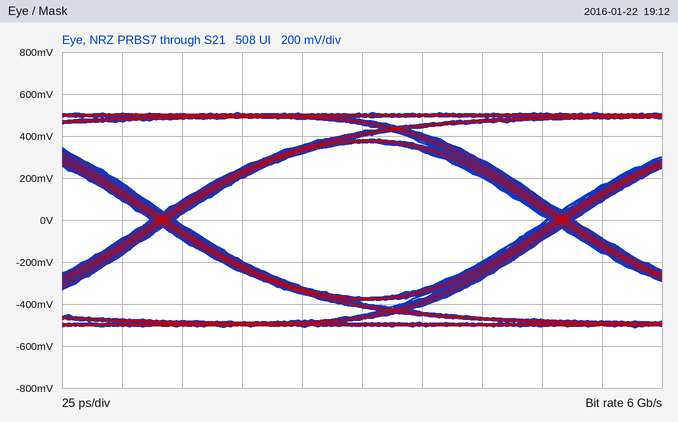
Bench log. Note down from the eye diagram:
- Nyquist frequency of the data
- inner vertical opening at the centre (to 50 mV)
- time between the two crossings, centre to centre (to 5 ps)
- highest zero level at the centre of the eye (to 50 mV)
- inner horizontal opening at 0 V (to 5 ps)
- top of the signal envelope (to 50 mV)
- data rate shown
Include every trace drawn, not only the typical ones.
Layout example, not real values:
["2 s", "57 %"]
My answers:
["3 GHz", "750 mV", "165 ps", "-350 mV", "155 ps", "500 mV", "6 Gb/s"]
